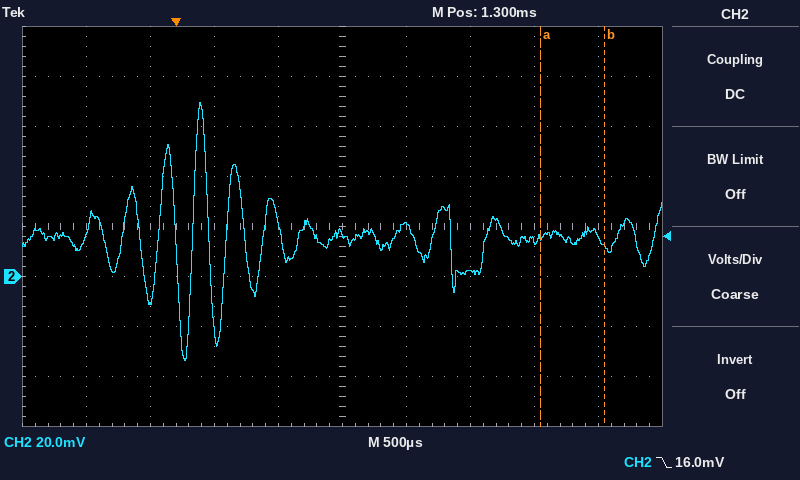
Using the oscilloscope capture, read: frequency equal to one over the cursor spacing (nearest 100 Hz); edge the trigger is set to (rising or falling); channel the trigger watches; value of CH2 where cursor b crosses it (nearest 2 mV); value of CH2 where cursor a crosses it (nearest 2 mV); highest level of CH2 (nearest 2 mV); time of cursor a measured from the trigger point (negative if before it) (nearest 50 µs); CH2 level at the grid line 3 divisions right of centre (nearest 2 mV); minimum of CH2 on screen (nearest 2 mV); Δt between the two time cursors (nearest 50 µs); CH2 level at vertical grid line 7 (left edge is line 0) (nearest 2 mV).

2.0 kHz
falling
CH2
12 mV
16 mV
70 mV
+2.85 ms
14 mV
-34 mV
500 µs
2 mV
